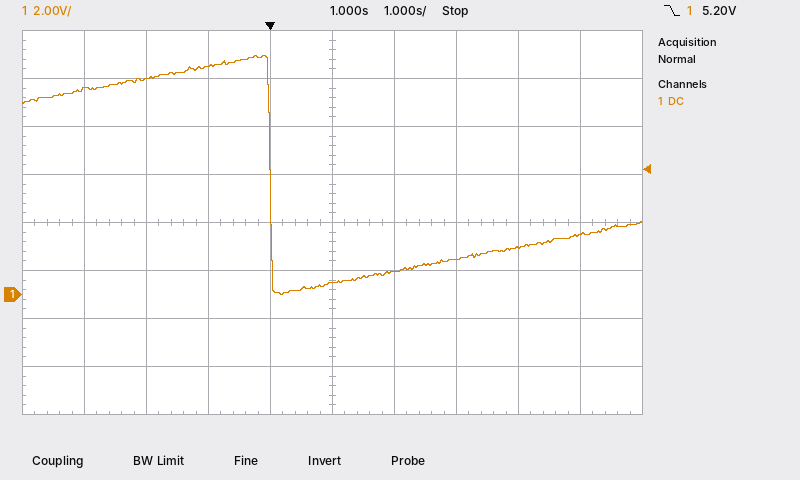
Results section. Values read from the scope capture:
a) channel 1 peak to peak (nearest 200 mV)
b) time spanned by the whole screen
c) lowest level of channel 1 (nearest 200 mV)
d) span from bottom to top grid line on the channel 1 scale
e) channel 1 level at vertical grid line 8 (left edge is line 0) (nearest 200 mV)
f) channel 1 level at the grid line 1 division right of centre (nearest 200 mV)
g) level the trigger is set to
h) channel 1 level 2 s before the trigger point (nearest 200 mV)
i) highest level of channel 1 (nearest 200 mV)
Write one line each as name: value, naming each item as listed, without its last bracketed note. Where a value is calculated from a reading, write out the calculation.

channel 1 peak to peak: 10.0 V − (0.0 V) = 10.0 V
time spanned by the whole screen: 10 s
lowest level of channel 1: 0.0 V
span from bottom to top grid line on the channel 1 scale: 16 V
channel 1 level at vertical grid line 8 (left edge is line 0): 2.0 V
channel 1 level at the grid line 1 division right of centre: 1.0 V
level the trigger is set to: 5.20 V
channel 1 level 2 s before the trigger point: 9.0 V
highest level of channel 1: 10.0 V
